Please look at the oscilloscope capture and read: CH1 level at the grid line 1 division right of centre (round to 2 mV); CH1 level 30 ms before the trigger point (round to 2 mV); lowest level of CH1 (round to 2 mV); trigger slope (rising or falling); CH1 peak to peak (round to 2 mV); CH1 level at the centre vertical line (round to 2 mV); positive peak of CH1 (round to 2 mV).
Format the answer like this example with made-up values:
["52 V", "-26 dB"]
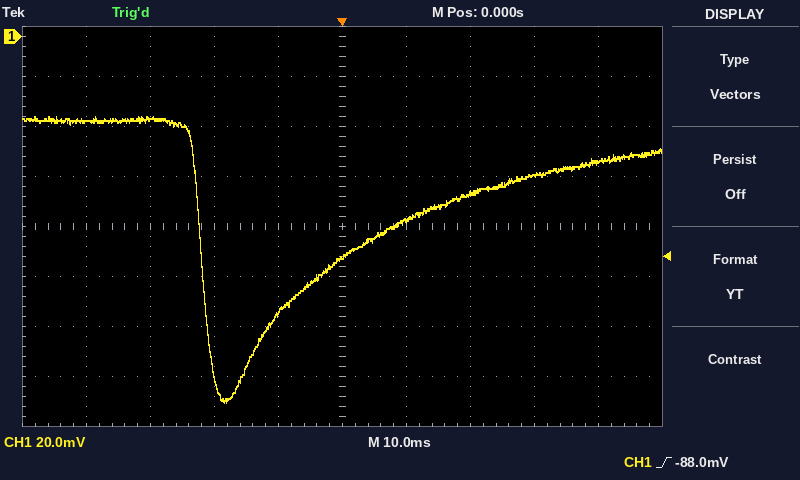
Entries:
["-74 mV", "-32 mV", "-146 mV", "rising", "114 mV", "-88 mV", "-32 mV"]
